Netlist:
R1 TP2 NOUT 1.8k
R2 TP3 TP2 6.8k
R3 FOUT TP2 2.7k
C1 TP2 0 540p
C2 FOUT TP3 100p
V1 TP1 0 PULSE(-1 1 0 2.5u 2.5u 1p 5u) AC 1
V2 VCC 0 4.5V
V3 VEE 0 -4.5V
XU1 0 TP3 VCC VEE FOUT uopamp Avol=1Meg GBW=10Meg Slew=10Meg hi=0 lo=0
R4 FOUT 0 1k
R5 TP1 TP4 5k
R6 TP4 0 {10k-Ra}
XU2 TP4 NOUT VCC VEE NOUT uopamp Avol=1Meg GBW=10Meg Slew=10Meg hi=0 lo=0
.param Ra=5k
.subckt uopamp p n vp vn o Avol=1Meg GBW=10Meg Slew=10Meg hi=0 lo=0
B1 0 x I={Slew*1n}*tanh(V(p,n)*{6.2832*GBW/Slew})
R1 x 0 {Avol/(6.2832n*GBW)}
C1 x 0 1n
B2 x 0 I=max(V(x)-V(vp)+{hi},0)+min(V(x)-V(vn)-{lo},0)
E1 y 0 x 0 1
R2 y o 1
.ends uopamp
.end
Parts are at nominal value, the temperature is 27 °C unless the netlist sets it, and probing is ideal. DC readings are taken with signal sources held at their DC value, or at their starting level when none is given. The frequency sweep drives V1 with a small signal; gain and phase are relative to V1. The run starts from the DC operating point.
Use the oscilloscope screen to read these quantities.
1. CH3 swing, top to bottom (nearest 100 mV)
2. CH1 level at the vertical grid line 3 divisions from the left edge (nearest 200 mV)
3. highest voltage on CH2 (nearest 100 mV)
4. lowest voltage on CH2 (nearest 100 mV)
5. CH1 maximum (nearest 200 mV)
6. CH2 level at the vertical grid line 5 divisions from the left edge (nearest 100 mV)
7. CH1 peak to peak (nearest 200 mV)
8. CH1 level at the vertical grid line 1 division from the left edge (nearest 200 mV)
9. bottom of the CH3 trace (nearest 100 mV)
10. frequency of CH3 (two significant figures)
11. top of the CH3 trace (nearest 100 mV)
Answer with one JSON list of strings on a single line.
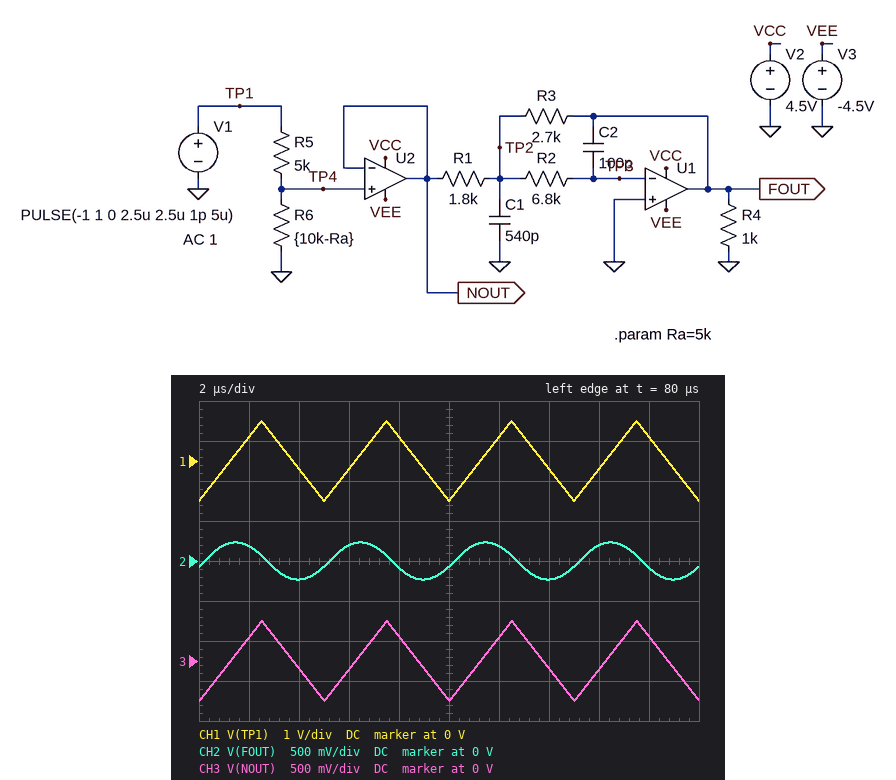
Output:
["1.0 V", "-200 mV", "200 mV", "-200 mV", "1.0 V", "-100 mV", "2.0 V", "600 mV", "-500 mV", "200 kHz", "500 mV"]
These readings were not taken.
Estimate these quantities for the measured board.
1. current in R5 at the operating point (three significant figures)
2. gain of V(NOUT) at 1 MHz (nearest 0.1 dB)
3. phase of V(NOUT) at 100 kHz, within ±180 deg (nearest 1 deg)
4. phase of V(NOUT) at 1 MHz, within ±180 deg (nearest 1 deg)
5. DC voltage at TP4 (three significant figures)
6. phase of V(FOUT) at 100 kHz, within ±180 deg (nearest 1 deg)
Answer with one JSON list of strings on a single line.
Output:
["100 µA", "-6.1 dB", "-1 deg", "-6 deg", "-500 mV", "114 deg"]
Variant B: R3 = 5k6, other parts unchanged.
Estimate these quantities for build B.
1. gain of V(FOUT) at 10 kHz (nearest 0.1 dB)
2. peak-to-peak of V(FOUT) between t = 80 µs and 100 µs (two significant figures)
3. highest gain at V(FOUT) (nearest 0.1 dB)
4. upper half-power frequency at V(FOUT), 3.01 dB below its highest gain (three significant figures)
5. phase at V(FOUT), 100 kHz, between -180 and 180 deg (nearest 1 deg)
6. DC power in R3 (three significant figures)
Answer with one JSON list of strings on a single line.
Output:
["3.7 dB", "510 mV", "3.8 dB", "56.5 kHz", "93 deg", "432 µW"]
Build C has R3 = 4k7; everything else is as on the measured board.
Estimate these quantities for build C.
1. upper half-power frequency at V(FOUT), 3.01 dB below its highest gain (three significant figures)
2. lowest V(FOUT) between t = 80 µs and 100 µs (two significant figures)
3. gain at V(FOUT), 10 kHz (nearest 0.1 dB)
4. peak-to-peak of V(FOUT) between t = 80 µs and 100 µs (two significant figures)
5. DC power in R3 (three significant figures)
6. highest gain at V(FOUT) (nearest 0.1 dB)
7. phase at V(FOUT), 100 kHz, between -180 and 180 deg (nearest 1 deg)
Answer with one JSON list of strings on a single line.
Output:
["66.0 kHz", "-250 mV", "2.2 dB", "500 mV", "363 µW", "2.3 dB", "98 deg"]
